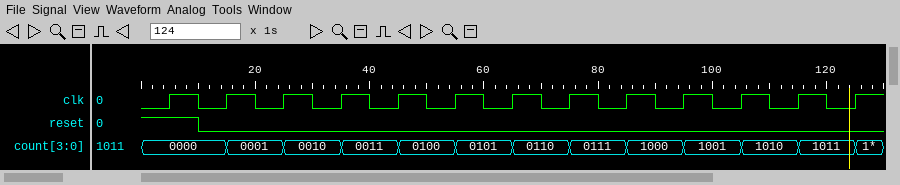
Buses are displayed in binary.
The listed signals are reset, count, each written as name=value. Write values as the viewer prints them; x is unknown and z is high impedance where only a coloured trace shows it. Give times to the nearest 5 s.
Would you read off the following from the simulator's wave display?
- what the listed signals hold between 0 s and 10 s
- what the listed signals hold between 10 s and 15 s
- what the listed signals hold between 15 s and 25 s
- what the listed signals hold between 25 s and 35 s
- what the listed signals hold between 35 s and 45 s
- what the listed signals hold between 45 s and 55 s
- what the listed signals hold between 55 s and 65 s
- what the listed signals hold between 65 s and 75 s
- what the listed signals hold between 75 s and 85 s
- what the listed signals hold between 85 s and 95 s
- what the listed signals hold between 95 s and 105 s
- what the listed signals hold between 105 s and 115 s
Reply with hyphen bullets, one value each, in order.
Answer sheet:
- reset=1, count=0000
- reset=0, count=0000
- reset=0, count=0001
- reset=0, count=0010
- reset=0, count=0011
- reset=0, count=0100
- reset=0, count=0101
- reset=0, count=0110
- reset=0, count=0111
- reset=0, count=1000
- reset=0, count=1001
- reset=0, count=1010
